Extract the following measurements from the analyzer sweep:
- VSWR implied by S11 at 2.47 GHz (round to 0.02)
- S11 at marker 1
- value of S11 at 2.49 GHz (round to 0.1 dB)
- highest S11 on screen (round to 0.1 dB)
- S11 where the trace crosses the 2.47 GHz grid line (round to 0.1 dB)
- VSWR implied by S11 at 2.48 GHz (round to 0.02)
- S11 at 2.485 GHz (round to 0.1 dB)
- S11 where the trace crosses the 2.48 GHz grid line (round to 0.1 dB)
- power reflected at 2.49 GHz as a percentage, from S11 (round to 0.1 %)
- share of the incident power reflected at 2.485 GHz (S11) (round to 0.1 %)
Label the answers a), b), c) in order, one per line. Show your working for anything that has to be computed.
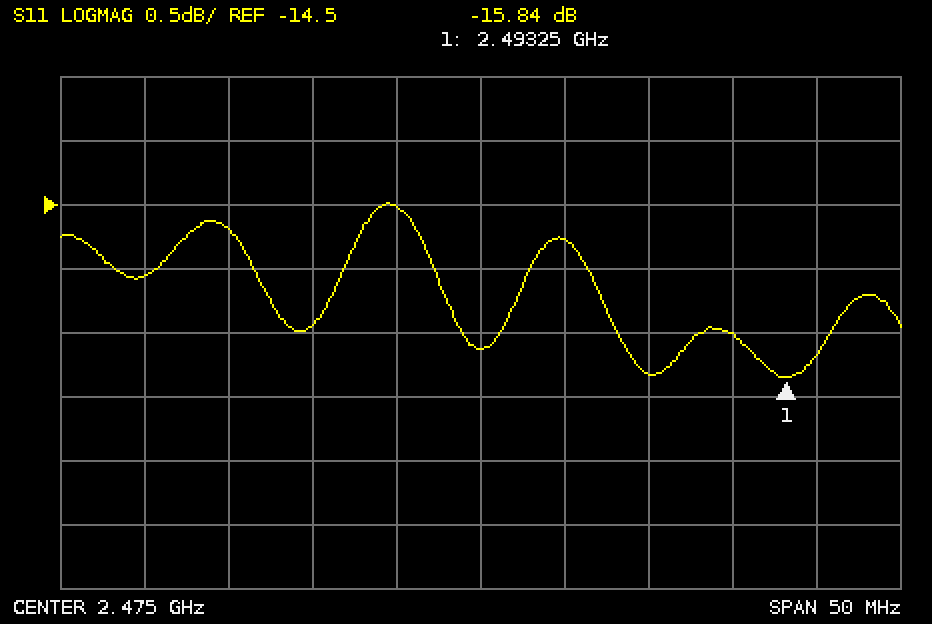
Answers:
a) |Γ| = 10^(-14.5/20) = 0.1884; VSWR = (1 + 0.1884)/(1 − 0.1884) ≈ 1.46
b) -15.84 dB
c) -15.5 dB
d) -14.5 dB
e) -14.5 dB
f) |Γ| = 10^(-14.8/20) = 0.1820; VSWR = (1 + 0.1820)/(1 − 0.1820) ≈ 1.44
g) -15.8 dB
h) -14.8 dB
i) 10^(-15.5/10) ≈ 2.8 %
j) 10^(-15.8/10) ≈ 2.6 %
